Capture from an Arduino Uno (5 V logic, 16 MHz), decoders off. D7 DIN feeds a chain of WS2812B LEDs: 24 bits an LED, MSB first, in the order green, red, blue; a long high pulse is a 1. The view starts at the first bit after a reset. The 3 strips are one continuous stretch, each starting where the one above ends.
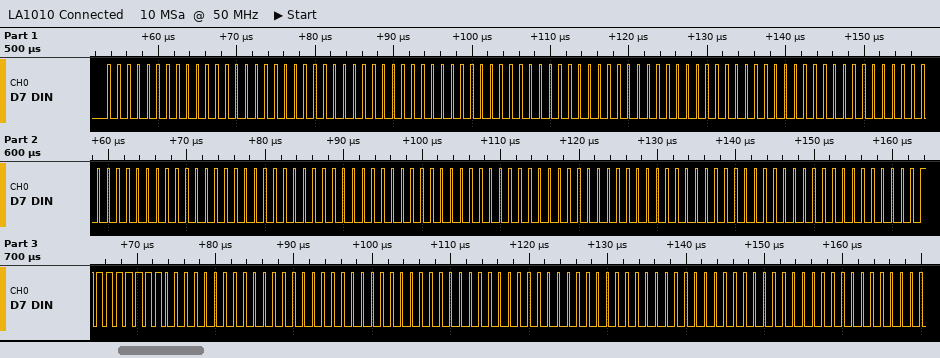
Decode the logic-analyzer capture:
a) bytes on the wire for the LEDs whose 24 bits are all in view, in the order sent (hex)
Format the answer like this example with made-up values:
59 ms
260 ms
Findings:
00 00 00 00 00 00 00 00 00 00 00 00 00 00 00 00 00 00 00 00 00 FF 00 00 00 00 00 00 00 00
